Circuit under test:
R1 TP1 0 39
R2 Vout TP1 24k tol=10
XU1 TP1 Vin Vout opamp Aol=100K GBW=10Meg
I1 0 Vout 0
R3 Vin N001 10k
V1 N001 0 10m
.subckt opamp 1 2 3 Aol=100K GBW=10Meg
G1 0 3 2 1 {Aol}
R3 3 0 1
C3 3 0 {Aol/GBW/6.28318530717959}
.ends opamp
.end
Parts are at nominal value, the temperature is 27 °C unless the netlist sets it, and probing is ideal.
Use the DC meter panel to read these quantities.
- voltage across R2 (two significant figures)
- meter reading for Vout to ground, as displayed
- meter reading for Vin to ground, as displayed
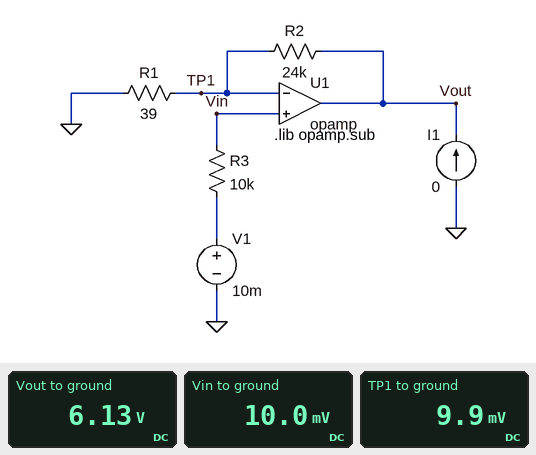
6.1 V
6.13 V
10.0 mV
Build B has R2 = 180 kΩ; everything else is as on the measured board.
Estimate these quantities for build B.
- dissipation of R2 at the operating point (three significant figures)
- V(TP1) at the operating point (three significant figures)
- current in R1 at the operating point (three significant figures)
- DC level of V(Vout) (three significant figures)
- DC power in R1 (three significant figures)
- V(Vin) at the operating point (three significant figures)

10.8 mW
9.56 mV
245 µA
44.1 V
2.34 µW
10.0 mV
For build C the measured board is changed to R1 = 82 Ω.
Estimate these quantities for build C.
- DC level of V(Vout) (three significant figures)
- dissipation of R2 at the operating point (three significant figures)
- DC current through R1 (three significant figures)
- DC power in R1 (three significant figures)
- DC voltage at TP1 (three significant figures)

2.93 V
355 µW
122 µA
1.21 µW
9.97 mV
